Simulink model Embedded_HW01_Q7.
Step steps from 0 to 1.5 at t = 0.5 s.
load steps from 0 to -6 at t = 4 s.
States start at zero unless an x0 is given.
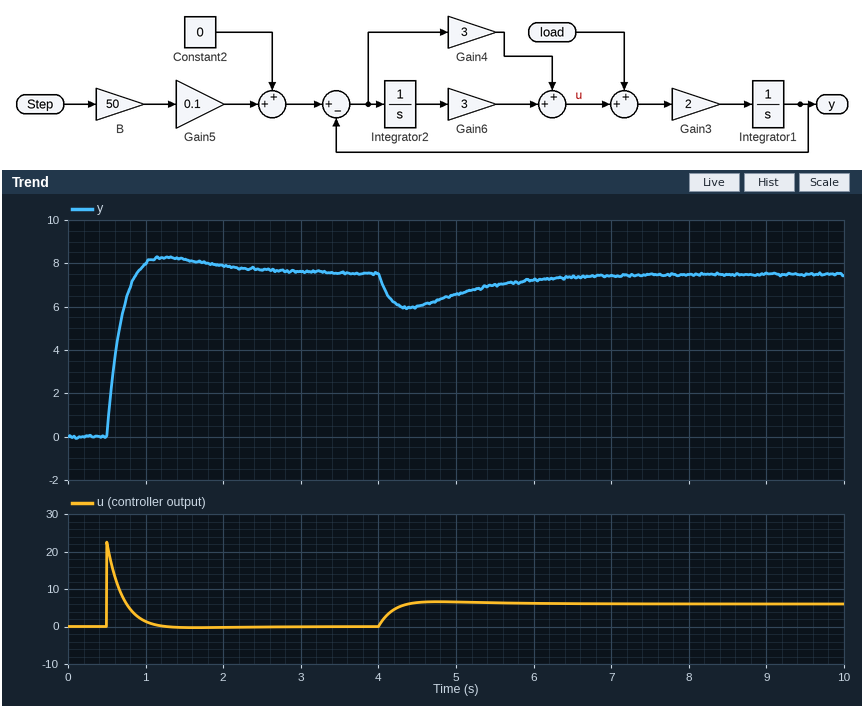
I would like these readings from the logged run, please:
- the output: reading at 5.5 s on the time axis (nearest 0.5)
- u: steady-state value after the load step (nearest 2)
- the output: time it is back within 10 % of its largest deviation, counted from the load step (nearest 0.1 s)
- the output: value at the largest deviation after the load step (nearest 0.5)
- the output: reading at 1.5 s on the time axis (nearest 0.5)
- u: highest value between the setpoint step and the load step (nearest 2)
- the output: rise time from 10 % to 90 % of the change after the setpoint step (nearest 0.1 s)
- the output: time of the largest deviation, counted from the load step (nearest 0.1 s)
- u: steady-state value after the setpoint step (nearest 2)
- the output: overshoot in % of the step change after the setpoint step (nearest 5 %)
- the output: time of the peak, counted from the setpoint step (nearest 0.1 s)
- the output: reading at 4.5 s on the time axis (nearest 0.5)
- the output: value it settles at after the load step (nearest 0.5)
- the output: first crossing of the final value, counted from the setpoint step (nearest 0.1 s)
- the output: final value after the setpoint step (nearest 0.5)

7.0
6
2.4 s
6.0
8.0
22
0.3 s
0.4 s
0
10 %
0.8 s
6.0
7.5
0.4 s
7.5
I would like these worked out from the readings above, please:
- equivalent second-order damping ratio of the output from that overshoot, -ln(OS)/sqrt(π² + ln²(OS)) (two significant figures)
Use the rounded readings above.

0.59
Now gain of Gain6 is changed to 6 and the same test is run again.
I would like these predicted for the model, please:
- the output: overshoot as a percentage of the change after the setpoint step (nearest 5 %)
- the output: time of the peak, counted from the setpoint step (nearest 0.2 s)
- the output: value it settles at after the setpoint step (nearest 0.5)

15 %
0.6 s
7.5
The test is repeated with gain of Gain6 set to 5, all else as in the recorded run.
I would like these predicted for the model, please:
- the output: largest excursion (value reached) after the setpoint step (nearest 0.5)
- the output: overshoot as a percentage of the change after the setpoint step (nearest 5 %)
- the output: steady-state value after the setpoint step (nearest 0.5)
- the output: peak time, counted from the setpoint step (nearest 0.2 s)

8.5
15 %
7.5
0.6 s
